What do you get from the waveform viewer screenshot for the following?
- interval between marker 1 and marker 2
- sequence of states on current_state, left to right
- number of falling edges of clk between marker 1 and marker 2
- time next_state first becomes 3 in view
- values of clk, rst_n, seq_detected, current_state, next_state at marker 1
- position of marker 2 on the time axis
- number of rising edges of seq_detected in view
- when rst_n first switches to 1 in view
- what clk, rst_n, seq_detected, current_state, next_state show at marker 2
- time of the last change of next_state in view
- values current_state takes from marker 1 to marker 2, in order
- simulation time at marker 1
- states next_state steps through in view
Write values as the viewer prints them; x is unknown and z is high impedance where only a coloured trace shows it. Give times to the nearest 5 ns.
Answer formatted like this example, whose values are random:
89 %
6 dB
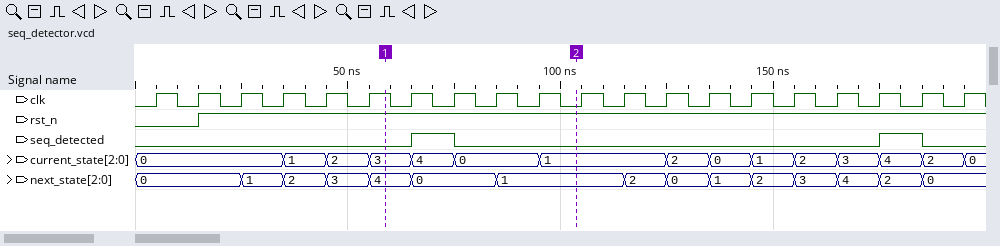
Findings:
45 ns
0, 1, 2, 3, 4, 0, 1, 2, 0, 1, 2, 3, 4, 2, 0
5
45 ns
clk=1, rst_n=1, seq_detected=0, current_state=3, next_state=4
105 ns
2
15 ns
clk=0, rst_n=1, seq_detected=0, current_state=1, next_state=1
185 ns
3, 4, 0, 1
60 ns
0, 1, 2, 3, 4, 0, 1, 2, 0, 1, 2, 3, 4, 2, 0
